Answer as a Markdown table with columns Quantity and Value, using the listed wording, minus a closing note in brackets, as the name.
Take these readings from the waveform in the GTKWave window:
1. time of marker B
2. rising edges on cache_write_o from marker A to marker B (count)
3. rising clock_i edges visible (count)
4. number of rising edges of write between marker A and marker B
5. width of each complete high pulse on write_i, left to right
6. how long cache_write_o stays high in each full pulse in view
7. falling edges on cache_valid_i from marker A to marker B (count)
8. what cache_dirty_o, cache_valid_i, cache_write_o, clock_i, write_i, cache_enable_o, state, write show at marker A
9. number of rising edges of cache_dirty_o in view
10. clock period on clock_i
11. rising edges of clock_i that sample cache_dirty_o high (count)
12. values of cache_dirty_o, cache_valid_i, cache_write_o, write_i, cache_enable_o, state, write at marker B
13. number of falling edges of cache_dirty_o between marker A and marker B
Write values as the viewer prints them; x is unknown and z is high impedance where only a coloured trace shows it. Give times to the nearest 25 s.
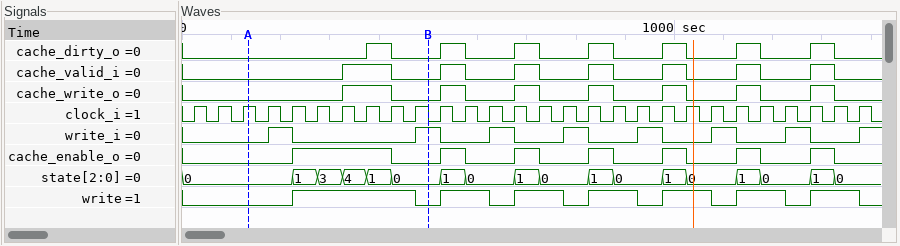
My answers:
| Quantity | Value |
|---|---|
| time of marker B | 500 s |
| rising edges on cache_write_o from marker A to marker B | 1 |
| rising clock_i edges visible | 28 |
| number of rising edges of write between marker A and marker B | 1 |
| width of each complete high pulse on write_i, left to right | 50 s, 50 s, 50 s, 50 s, 50 s, 50 s, 50 s |
| how long cache_write_o stays high in each full pulse in view | 100 s, 50 s, 50 s, 50 s, 50 s, 50 s, 50 s |
| falling edges on cache_valid_i from marker A to marker B | 1 |
| what cache_dirty_o, cache_valid_i, cache_write_o, clock_i, write_i, cache_enable_o, state, write show at marker A | cache_dirty_o=0, cache_valid_i=0, cache_write_o=0, clock_i=1, write_i=0, cache_enable_o=0, state=0, write=0 |
| number of rising edges of cache_dirty_o in view | 7 |
| clock period on clock_i | 50 s |
| rising edges of clock_i that sample cache_dirty_o high | 7 |
| values of cache_dirty_o, cache_valid_i, cache_write_o, write_i, cache_enable_o, state, write at marker B | cache_dirty_o=0, cache_valid_i=0, cache_write_o=0, write_i=1, cache_enable_o=0, state=0, write=0 |
| number of falling edges of cache_dirty_o between marker A and marker B | 1 |
